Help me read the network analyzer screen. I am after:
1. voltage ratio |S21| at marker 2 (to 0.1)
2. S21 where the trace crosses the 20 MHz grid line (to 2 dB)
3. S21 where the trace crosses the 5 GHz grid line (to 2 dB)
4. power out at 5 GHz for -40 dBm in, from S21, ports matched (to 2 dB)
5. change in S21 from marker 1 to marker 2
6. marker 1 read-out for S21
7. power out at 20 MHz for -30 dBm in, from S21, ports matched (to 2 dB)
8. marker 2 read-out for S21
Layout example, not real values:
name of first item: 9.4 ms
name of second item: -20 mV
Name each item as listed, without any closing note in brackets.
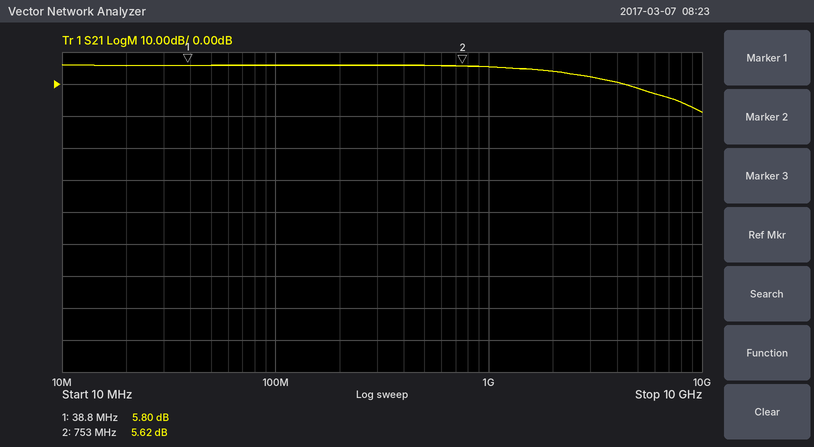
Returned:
voltage ratio |S21| at marker 2: 1.9
S21 where the trace crosses the 20 MHz grid line: 6 dB
S21 where the trace crosses the 5 GHz grid line: -2 dB
power out at 5 GHz for -40 dBm in, from S21, ports matched: -42 dBm
change in S21 from marker 1 to marker 2: -0.18 dB
marker 1 read-out for S21: 5.80 dB
power out at 20 MHz for -30 dBm in, from S21, ports matched: -24 dBm
marker 2 read-out for S21: 5.62 dB
